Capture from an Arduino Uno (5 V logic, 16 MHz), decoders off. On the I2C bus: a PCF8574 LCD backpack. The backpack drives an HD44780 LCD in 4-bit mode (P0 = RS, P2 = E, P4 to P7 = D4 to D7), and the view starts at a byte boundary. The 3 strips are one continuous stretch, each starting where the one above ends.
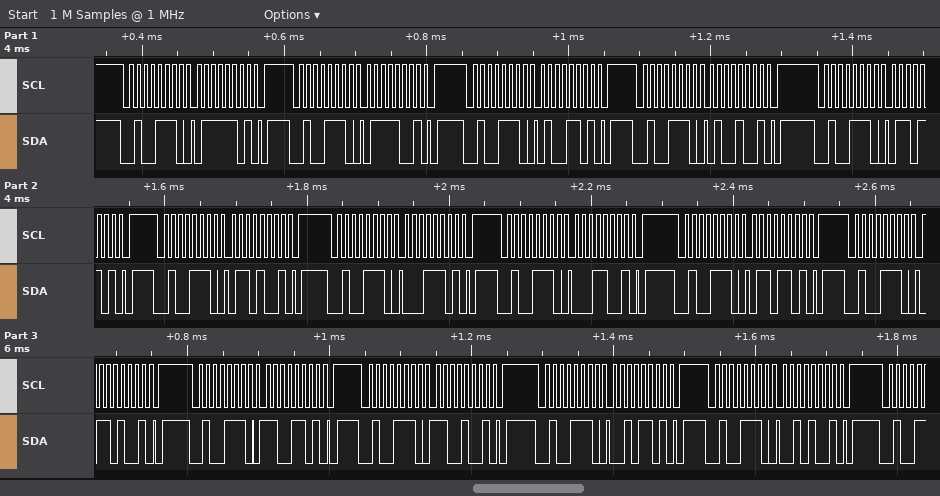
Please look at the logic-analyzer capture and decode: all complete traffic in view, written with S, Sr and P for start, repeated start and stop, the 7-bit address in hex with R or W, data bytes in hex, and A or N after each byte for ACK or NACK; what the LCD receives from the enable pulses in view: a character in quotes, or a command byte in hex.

S 27W A 7D A P S 27W A 79 A P S 27W A 4D A P S 27W A 49 A P S 27W A 6D A P S 27W A 69 A P S 27W A 1D A P S 27W A 19 A P S 27W A 6D A P S 27W A 69 A P S 27W A CD A P S 27W A C9 A P S 27W A 2D A P S 27W A 29 A P
't' 'a' 'l'
